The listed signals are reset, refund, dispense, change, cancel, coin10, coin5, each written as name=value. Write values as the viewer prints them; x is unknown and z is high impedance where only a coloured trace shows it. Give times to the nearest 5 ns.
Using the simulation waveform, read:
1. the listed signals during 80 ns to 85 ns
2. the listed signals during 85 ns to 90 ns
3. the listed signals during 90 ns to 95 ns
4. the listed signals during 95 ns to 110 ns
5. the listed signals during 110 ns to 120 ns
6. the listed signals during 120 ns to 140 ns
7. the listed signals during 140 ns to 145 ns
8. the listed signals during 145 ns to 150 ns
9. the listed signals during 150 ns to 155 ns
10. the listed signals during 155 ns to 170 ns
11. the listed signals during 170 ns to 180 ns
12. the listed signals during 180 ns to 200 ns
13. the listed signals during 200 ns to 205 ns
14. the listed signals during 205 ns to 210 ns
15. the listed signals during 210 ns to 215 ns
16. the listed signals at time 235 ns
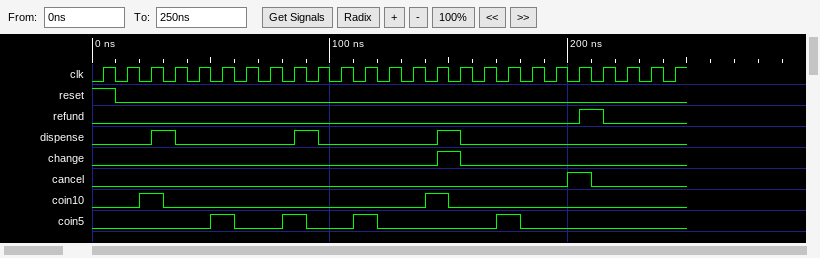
reset=0, refund=0, dispense=0, change=0, cancel=0, coin10=0, coin5=1
reset=0, refund=0, dispense=1, change=0, cancel=0, coin10=0, coin5=1
reset=0, refund=0, dispense=1, change=0, cancel=0, coin10=0, coin5=0
reset=0, refund=0, dispense=0, change=0, cancel=0, coin10=0, coin5=0
reset=0, refund=0, dispense=0, change=0, cancel=0, coin10=0, coin5=1
reset=0, refund=0, dispense=0, change=0, cancel=0, coin10=0, coin5=0
reset=0, refund=0, dispense=0, change=0, cancel=0, coin10=1, coin5=0
reset=0, refund=0, dispense=1, change=1, cancel=0, coin10=1, coin5=0
reset=0, refund=0, dispense=1, change=1, cancel=0, coin10=0, coin5=0
reset=0, refund=0, dispense=0, change=0, cancel=0, coin10=0, coin5=0
reset=0, refund=0, dispense=0, change=0, cancel=0, coin10=0, coin5=1
reset=0, refund=0, dispense=0, change=0, cancel=0, coin10=0, coin5=0
reset=0, refund=0, dispense=0, change=0, cancel=1, coin10=0, coin5=0
reset=0, refund=1, dispense=0, change=0, cancel=1, coin10=0, coin5=0
reset=0, refund=1, dispense=0, change=0, cancel=0, coin10=0, coin5=0
reset=0, refund=0, dispense=0, change=0, cancel=0, coin10=0, coin5=0
